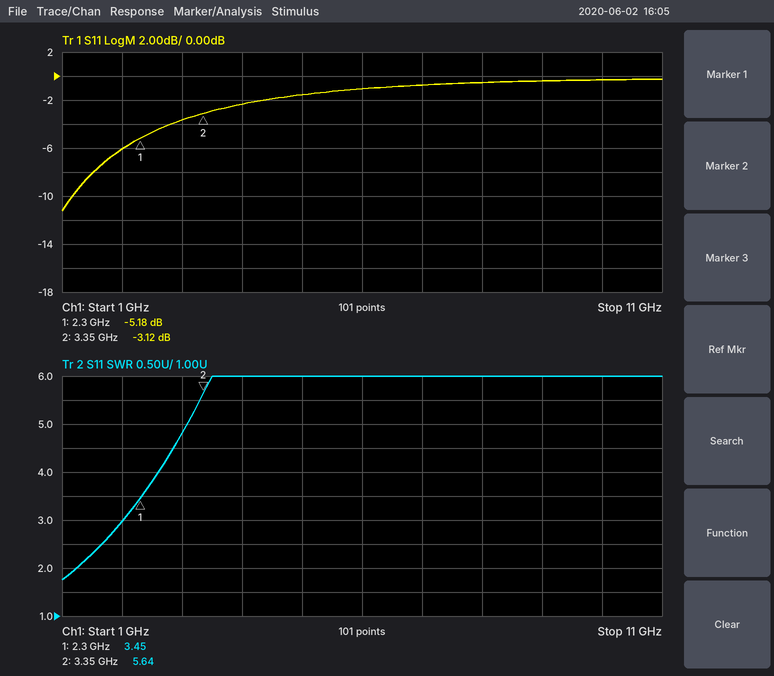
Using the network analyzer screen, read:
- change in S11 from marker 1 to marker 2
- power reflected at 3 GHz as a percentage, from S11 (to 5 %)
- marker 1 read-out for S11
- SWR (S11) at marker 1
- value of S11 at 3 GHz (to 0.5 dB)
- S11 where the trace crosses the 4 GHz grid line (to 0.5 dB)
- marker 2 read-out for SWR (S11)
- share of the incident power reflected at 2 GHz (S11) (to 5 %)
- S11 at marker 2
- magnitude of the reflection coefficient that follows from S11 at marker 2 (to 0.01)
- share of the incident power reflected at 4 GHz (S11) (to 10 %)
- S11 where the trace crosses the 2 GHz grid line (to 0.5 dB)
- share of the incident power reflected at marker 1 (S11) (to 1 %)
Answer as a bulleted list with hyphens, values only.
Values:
- 2.06 dB
- 45 %
- -5.18 dB
- 3.45
- -3.5 dB
- -2.5 dB
- 5.64
- 25 %
- -3.12 dB
- 0.70
- 60 %
- -6.0 dB
- 30 %
